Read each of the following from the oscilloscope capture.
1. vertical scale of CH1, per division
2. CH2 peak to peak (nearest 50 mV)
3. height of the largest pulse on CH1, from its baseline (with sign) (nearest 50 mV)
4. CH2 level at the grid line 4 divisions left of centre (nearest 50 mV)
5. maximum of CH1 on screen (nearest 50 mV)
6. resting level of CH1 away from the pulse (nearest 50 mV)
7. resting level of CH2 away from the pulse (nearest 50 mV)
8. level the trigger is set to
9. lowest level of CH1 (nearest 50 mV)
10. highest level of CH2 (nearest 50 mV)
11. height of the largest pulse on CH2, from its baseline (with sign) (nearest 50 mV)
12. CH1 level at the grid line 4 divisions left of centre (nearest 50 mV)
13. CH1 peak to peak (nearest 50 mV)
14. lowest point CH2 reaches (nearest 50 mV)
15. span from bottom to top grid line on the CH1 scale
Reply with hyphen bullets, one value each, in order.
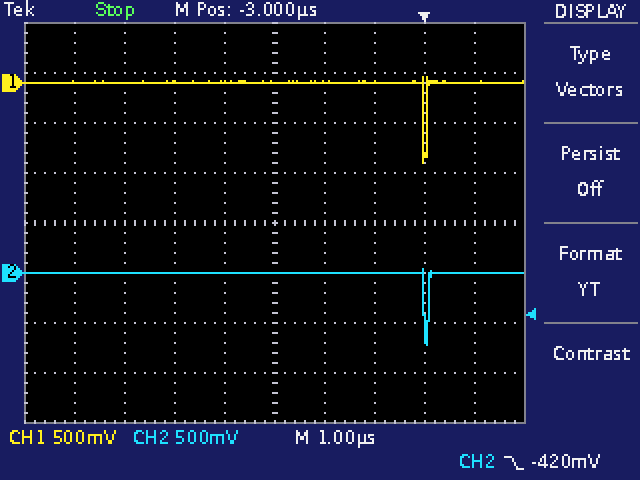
- 500 mV
- 750 mV
- -800 mV
- 0 mV
- 50 mV
- 0 mV
- 0 mV
- -420 mV
- -800 mV
- 50 mV
- -700 mV
- 0 mV
- 850 mV
- -700 mV
- 4 V
